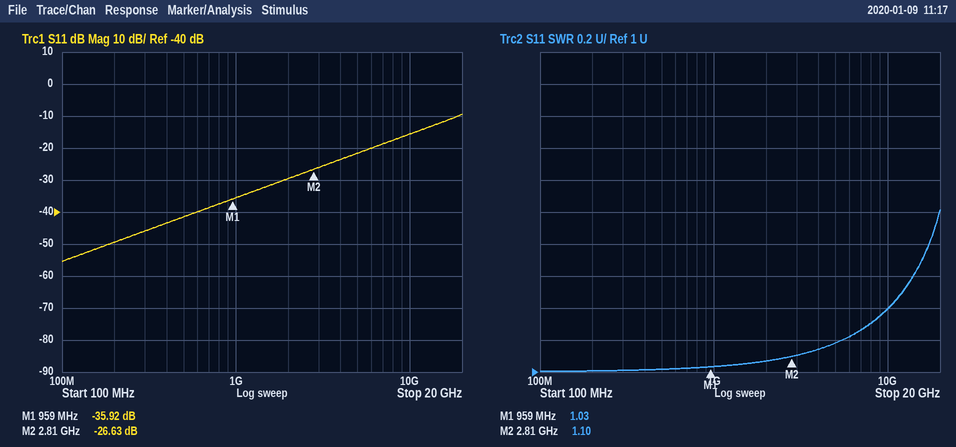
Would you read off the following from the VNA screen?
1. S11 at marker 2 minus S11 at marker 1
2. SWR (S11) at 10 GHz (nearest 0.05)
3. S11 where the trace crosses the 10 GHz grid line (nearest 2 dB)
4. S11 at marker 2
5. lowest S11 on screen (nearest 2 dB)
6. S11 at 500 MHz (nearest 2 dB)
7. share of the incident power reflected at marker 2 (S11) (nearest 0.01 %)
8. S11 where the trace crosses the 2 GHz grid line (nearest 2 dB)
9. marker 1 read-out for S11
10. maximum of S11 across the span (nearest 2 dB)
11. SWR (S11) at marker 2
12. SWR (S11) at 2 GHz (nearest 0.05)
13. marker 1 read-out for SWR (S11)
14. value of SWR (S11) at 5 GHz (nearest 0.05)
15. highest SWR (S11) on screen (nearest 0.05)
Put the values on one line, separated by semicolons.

9.29 dB; 1.40; -16 dB; -26.63 dB; -56 dB; -42 dB; 0.22 %; -30 dB; -35.92 dB; -10 dB; 1.10; 1.05; 1.03; 1.20; 2.00
